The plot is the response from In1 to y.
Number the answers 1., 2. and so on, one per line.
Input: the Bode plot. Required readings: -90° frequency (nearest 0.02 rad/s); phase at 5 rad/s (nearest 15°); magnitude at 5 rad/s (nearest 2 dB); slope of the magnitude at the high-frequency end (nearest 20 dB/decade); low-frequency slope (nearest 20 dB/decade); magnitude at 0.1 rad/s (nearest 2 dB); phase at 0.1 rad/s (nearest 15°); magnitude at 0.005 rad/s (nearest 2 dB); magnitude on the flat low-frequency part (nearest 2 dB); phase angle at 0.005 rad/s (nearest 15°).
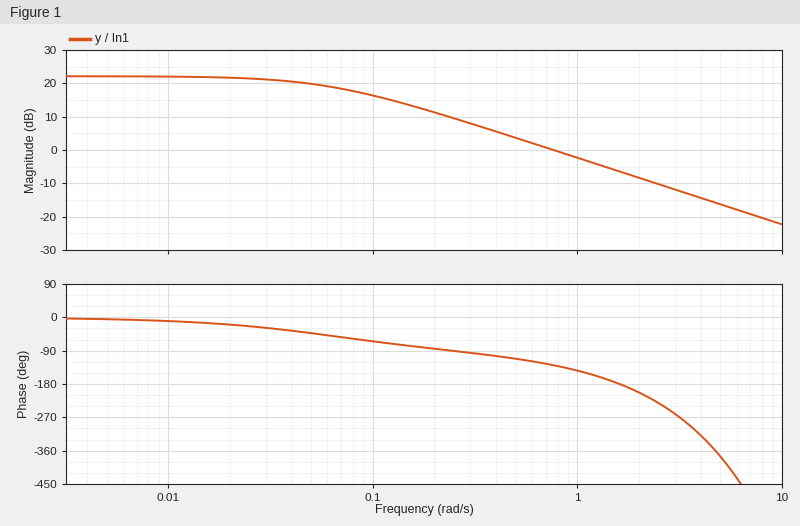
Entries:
1. 0.24 rad/s
2. -375°
3. -16 dB
4. -20 dB/decade
5. 0 dB/decade
6. 16 dB
7. -60°
8. 22 dB
9. 22 dB
10. 0°
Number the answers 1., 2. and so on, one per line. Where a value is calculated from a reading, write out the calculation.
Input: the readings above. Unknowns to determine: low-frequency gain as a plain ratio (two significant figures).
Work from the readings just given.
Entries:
1. 10^(22 / 20) = 13
